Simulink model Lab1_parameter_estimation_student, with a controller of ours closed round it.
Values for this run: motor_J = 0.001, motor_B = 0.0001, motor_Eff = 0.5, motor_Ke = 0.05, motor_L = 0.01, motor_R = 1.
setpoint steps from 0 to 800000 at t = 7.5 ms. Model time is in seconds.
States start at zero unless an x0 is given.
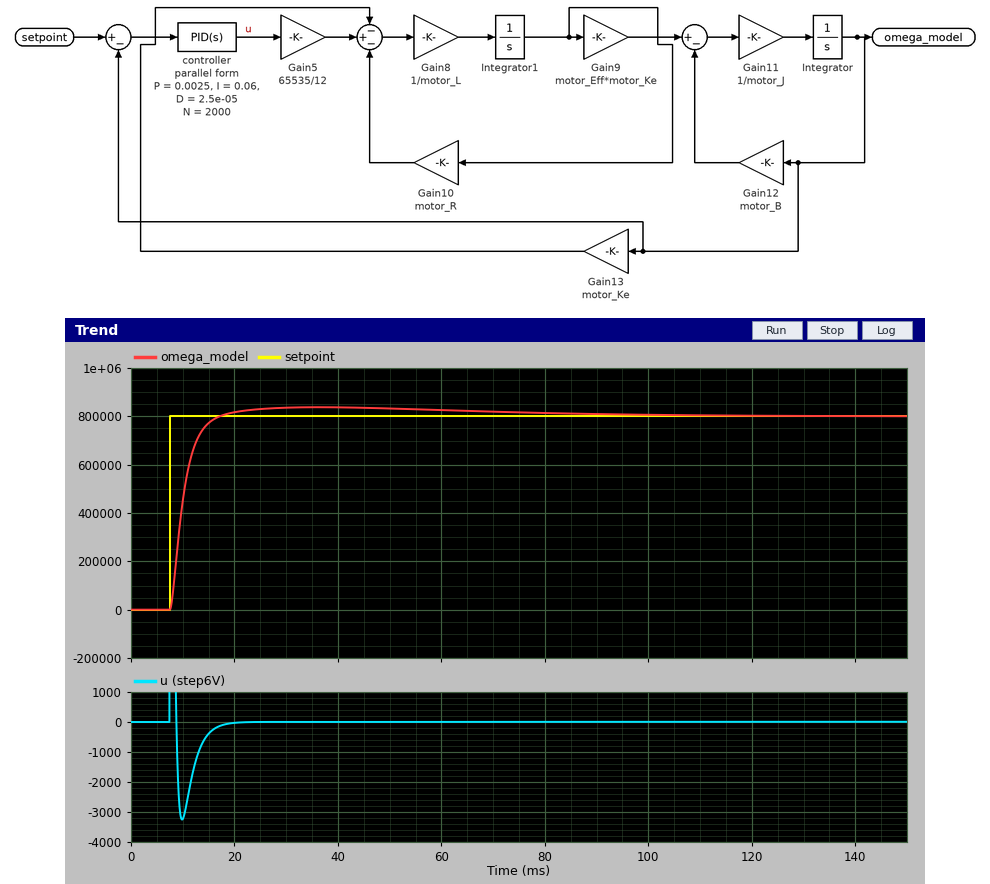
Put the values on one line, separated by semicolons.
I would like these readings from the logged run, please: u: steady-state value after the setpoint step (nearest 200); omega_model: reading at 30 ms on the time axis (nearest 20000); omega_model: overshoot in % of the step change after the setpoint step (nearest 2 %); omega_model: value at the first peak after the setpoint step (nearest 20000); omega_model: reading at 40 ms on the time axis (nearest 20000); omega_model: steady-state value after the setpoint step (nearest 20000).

0; 840000; 4 %; 840000; 840000; 800000
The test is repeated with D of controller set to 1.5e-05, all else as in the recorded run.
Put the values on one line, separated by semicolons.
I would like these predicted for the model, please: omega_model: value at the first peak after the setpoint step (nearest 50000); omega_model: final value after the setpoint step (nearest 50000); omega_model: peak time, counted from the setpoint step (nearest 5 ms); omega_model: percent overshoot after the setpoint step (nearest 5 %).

900000; 800000; 15 ms; 10 %
